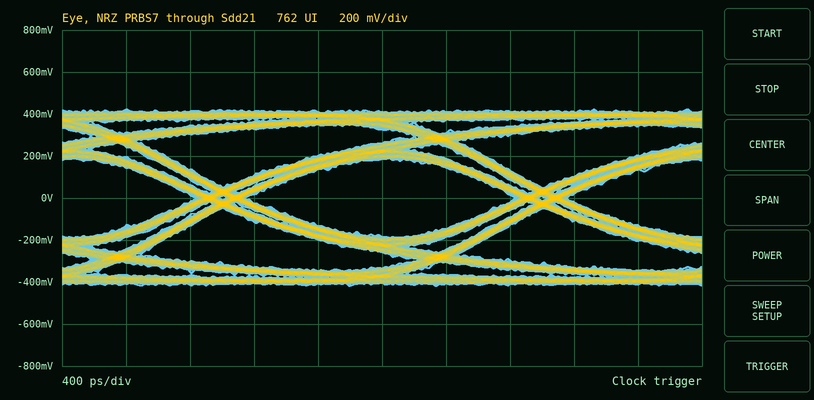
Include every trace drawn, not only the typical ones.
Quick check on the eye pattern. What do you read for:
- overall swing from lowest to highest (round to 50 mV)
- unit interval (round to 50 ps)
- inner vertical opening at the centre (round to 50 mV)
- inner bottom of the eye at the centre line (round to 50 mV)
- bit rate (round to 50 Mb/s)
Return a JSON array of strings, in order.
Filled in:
["850 mV", "2.00 ns", "350 mV", "-200 mV", "500 Mb/s"]
